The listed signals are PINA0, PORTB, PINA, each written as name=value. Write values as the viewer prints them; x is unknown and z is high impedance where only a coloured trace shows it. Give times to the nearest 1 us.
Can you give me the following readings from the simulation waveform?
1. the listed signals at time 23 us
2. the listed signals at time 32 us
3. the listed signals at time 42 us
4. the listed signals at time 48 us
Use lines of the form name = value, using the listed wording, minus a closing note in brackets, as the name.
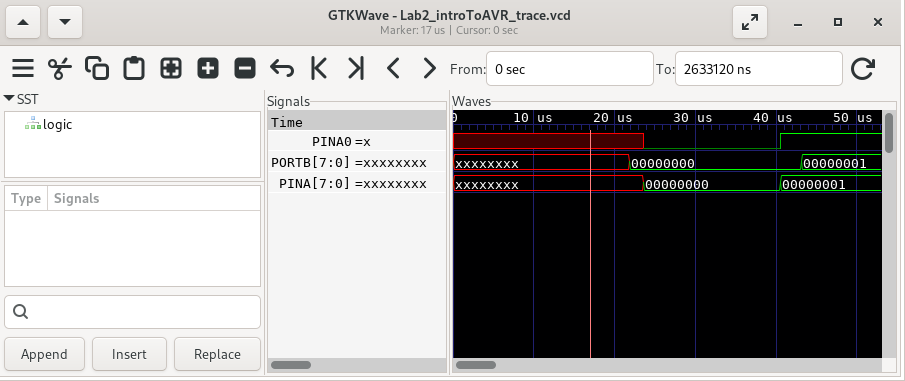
the listed signals at time 23 us = PINA0=x, PORTB=00000000, PINA=xxxxxxxx
the listed signals at time 32 us = PINA0=0, PORTB=00000000, PINA=00000000
the listed signals at time 42 us = PINA0=1, PORTB=00000000, PINA=00000001
the listed signals at time 48 us = PINA0=1, PORTB=00000001, PINA=00000001
